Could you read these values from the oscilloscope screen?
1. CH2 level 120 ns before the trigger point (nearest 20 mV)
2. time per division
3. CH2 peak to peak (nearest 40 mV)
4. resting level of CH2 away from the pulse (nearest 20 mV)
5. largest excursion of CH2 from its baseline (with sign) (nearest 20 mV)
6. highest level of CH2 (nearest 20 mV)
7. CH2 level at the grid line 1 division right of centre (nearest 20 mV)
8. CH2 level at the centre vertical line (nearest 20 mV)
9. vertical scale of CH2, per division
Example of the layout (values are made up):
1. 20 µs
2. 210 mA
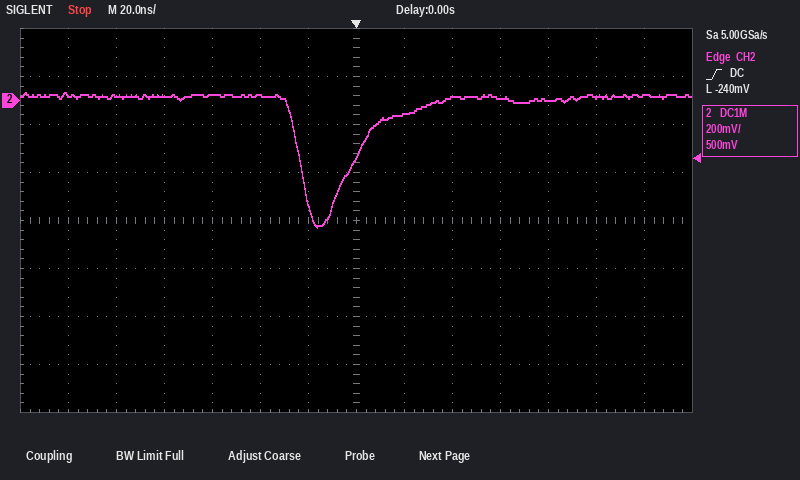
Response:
1. 20 mV
2. 20 ns
3. 560 mV
4. 20 mV
5. -540 mV
6. 40 mV
7. -60 mV
8. -240 mV
9. 200 mV
